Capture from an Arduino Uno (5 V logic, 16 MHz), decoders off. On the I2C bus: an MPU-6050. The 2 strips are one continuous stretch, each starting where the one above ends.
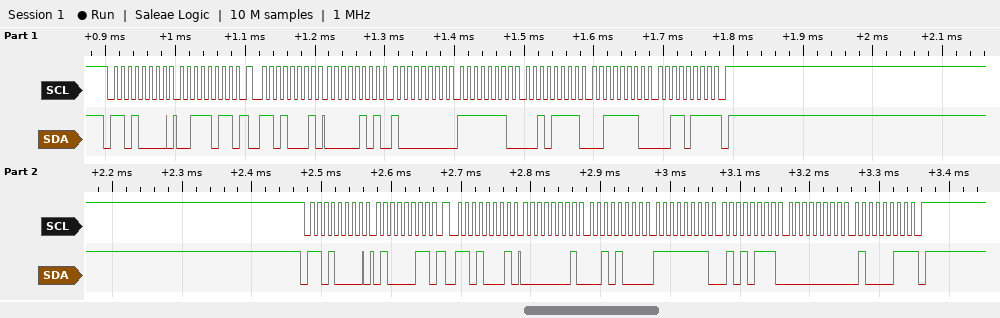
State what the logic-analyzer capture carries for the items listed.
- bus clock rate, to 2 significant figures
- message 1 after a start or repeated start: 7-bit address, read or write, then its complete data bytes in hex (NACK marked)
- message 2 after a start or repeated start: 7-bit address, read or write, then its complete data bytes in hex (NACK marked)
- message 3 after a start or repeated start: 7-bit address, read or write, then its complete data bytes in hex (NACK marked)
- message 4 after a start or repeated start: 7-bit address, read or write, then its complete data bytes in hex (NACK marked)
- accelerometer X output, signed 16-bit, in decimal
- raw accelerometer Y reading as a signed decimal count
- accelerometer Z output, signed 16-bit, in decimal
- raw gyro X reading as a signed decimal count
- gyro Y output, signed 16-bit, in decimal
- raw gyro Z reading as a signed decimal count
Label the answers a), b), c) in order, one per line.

a) 100 kHz
b) 0x68 write: 3B
c) 0x68 read: 05 80 FE 2F 3E 37 NACK
d) 0x68 write: 43
e) 0x68 read: 01 28 FF 57 00 43 NACK
f) 1408
g) -465
h) 15927
i) 296
j) -169
k) 67
